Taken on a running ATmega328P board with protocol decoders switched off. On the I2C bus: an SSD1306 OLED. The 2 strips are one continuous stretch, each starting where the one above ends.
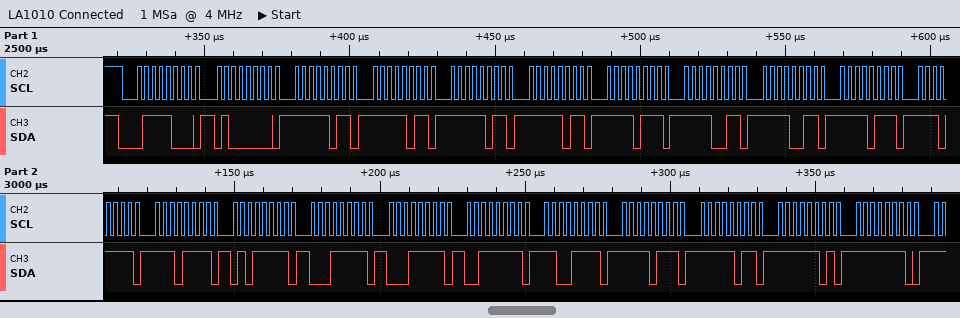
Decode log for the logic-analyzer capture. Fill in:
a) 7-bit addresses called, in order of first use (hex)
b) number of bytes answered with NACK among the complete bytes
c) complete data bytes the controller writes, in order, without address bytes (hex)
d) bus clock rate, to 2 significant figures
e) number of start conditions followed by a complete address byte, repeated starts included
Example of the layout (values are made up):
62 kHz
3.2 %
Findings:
0x3C
0
40 FB FB FB FB F7 F3 F3 F7 EF EF 5F 1F 1F 3F CF F7 FB FD FE
400 kHz
1
